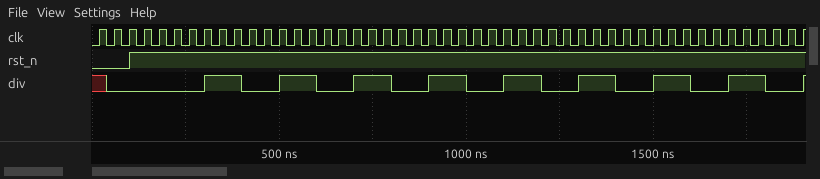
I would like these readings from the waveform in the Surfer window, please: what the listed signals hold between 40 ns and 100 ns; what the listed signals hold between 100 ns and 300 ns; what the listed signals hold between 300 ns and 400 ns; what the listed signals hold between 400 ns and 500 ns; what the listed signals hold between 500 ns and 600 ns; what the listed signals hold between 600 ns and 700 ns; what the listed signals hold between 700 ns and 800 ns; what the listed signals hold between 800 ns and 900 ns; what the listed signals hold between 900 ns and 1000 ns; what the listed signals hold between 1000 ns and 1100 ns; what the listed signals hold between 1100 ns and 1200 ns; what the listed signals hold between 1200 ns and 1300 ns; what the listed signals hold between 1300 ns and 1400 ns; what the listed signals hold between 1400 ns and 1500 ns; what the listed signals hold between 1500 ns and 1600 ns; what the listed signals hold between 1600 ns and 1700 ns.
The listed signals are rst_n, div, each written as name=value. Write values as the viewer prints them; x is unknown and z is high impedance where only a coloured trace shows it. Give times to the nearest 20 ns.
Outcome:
rst_n=0, div=0
rst_n=1, div=0
rst_n=1, div=1
rst_n=1, div=0
rst_n=1, div=1
rst_n=1, div=0
rst_n=1, div=1
rst_n=1, div=0
rst_n=1, div=1
rst_n=1, div=0
rst_n=1, div=1
rst_n=1, div=0
rst_n=1, div=1
rst_n=1, div=0
rst_n=1, div=1
rst_n=1, div=0
